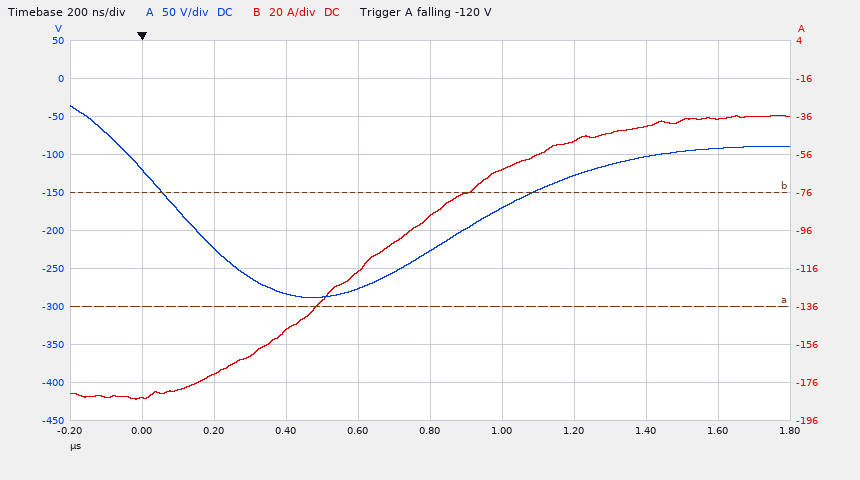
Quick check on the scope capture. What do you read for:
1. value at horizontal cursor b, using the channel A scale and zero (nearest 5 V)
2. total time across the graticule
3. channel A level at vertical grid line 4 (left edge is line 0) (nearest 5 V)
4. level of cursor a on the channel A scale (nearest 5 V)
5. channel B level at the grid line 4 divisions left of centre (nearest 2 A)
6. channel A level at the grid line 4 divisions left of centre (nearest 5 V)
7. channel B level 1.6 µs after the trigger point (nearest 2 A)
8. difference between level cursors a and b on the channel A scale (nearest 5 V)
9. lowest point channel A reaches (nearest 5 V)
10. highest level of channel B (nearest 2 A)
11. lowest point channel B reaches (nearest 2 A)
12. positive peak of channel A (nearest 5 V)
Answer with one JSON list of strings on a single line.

["-150 V", "2 µs", "-275 V", "-300 V", "-184 A", "-120 V", "-38 A", "150 V", "-290 V", "-36 A", "-184 A", "-35 V"]
